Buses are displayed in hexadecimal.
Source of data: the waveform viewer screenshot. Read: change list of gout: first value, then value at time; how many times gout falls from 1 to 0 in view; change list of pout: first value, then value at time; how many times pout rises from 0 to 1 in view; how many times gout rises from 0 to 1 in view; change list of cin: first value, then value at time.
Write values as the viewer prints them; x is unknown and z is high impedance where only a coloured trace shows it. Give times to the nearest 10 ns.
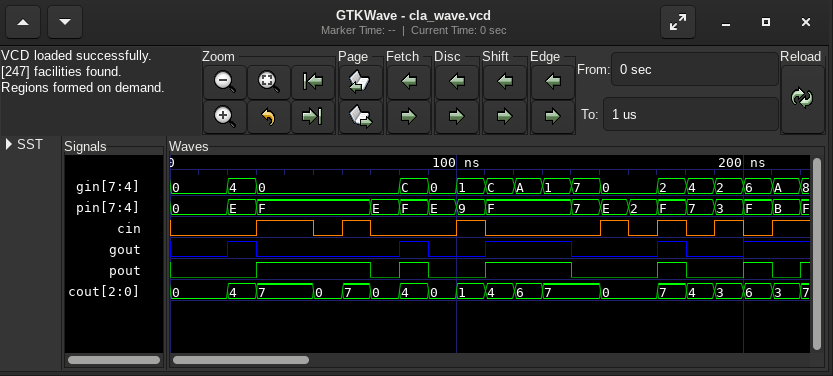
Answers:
0, 1 at 20 ns, 0 at 30 ns, 1 at 80 ns, 0 at 90 ns, 1 at 110 ns, 0 at 140 ns, 1 at 170 ns, 0 at 180 ns, 1 at 200 ns
4
0, 1 at 30 ns, 0 at 70 ns, 1 at 80 ns, 0 at 90 ns, 1 at 110 ns, 0 at 140 ns, 1 at 170 ns, 0 at 180 ns, 1 at 200 ns, 0 at 210 ns, 1 at 220 ns
6
5
0, 1 at 30 ns, 0 at 50 ns, 1 at 60 ns, 0 at 70 ns, 1 at 100 ns, 0 at 110 ns, 1 at 150 ns, 0 at 160 ns, 1 at 170 ns, 0 at 180 ns, 1 at 190 ns, 0 at 200 ns, 1 at 210 ns
